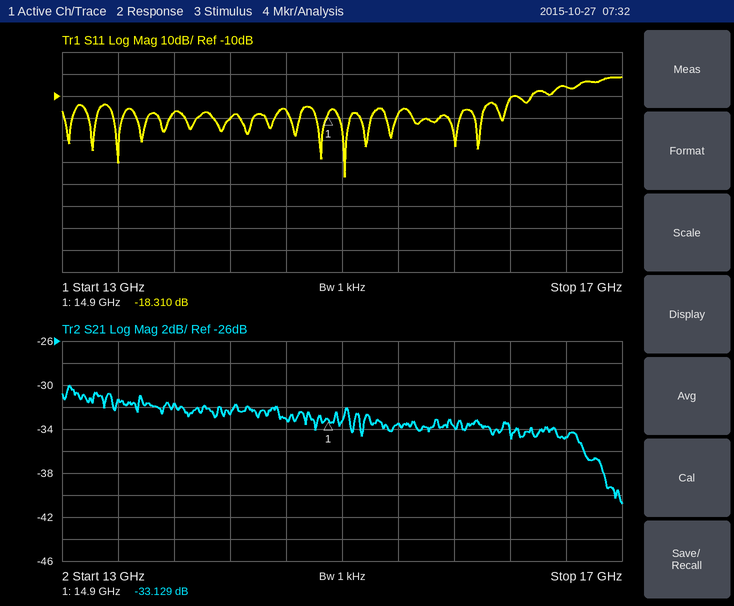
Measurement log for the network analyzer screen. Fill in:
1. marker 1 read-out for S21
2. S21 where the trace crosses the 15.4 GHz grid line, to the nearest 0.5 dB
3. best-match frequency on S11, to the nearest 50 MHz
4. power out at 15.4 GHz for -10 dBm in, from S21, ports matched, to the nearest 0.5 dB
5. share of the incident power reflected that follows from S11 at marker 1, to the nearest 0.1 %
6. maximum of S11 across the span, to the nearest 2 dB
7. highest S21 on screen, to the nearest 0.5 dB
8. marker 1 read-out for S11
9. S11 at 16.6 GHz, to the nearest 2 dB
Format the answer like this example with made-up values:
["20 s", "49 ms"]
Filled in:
["-33.129 dB", "-33.5 dB", "15.00 GHz", "-43.5 dBm", "1.5 %", "-2 dB", "-30.0 dB", "-18.310 dB", "-6 dB"]
